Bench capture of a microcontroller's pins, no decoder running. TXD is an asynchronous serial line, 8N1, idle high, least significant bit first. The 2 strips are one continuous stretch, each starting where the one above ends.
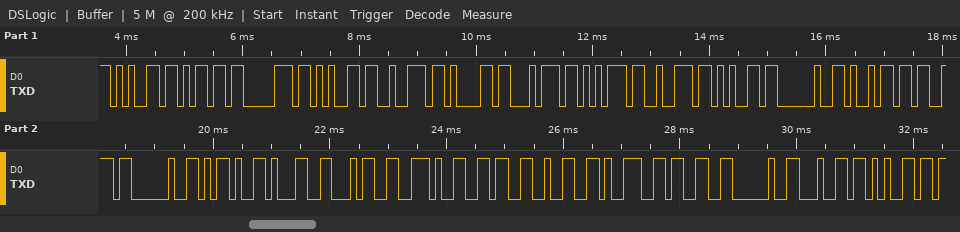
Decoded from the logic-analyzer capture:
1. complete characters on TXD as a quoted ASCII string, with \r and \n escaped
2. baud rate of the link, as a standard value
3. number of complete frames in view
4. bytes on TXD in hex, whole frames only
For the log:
"emperature is -14.6293 de"
9600 baud
25
65 6D 70 65 72 61 74 75 72 65 20 69 73 20 2D 31 34 2E 36 32 39 33 20 64 65
